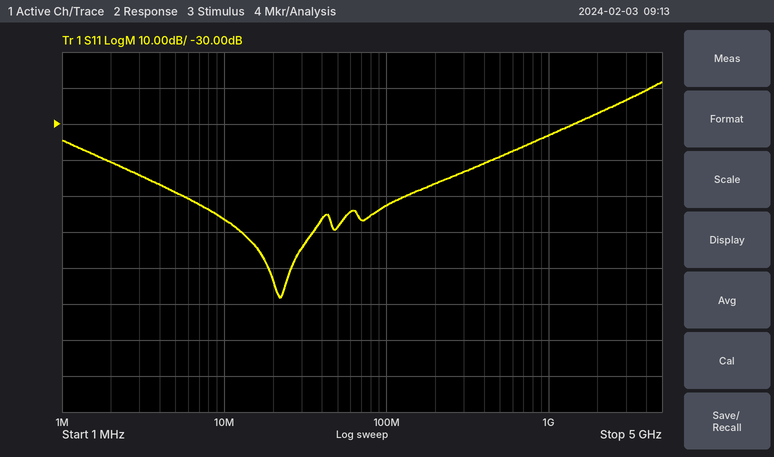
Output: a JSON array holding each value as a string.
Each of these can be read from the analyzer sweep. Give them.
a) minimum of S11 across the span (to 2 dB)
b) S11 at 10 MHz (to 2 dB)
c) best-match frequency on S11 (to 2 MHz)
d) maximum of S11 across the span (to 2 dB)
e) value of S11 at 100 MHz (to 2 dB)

["-78 dB", "-56 dB", "22 MHz", "-18 dB", "-52 dB"]
